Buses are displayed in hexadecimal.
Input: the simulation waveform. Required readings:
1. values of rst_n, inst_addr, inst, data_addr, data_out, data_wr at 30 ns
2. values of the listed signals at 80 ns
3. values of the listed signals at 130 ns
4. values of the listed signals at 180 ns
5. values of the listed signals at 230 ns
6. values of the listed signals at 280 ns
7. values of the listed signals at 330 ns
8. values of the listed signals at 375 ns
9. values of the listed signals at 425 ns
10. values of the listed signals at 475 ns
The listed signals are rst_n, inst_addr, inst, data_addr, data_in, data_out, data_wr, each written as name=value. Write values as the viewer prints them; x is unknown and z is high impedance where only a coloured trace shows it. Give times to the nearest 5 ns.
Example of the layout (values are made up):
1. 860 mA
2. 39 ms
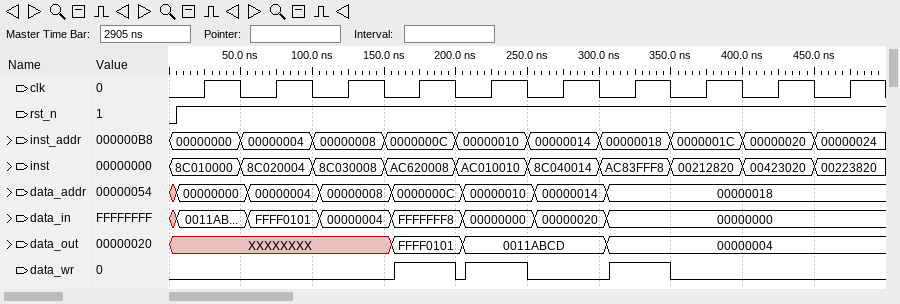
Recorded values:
1. rst_n=1, inst_addr=00000000, inst=8C010000, data_addr=00000000, data_out=XXXXXXXX, data_wr=0
2. rst_n=1, inst_addr=00000004, inst=8C020004, data_addr=00000004, data_in=FFFF0101, data_out=XXXXXXXX, data_wr=0
3. rst_n=1, inst_addr=00000008, inst=8C030008, data_addr=00000008, data_in=00000004, data_out=XXXXXXXX, data_wr=0
4. rst_n=1, inst_addr=0000000C, inst=AC620008, data_addr=0000000C, data_in=FFFFFFF8, data_out=FFFF0101, data_wr=1
5. rst_n=1, inst_addr=00000010, inst=AC010010, data_addr=00000010, data_in=00000000, data_out=0011ABCD, data_wr=1
6. rst_n=1, inst_addr=00000014, inst=8C040014, data_addr=00000014, data_in=00000020, data_out=0011ABCD, data_wr=0
7. rst_n=1, inst_addr=00000018, inst=AC83FFF8, data_addr=00000018, data_in=00000000, data_out=00000004, data_wr=1
8. rst_n=1, inst_addr=0000001C, inst=00212820, data_addr=00000018, data_in=00000000, data_out=00000004, data_wr=0
9. rst_n=1, inst_addr=00000020, inst=00423020, data_addr=00000018, data_in=00000000, data_out=00000004, data_wr=0
10. rst_n=1, inst_addr=00000024, inst=00223820, data_addr=00000018, data_in=00000000, data_out=00000004, data_wr=0
